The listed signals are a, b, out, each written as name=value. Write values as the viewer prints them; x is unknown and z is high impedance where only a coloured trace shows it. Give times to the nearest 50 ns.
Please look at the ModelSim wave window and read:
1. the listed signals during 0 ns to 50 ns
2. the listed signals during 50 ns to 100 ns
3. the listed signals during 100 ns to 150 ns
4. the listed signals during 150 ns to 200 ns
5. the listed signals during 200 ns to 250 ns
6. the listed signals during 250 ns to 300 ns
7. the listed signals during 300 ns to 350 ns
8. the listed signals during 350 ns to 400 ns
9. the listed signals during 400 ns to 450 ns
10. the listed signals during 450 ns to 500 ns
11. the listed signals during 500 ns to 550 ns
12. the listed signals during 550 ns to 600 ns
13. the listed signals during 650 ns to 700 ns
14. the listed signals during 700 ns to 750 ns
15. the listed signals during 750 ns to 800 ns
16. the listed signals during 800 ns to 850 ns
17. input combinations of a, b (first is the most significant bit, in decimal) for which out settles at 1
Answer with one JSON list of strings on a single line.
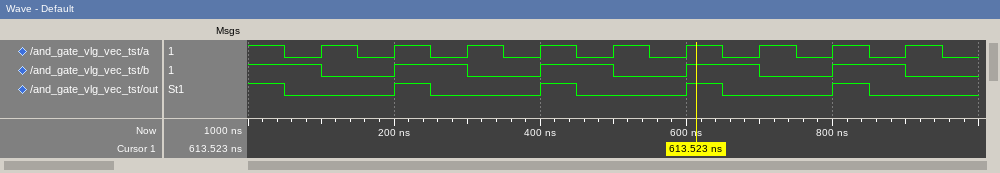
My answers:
["a=1, b=1, out=1", "a=0, b=1, out=0", "a=1, b=0, out=0", "a=0, b=0, out=0", "a=1, b=1, out=1", "a=0, b=1, out=0", "a=1, b=0, out=0", "a=0, b=0, out=0", "a=1, b=1, out=1", "a=0, b=1, out=0", "a=1, b=0, out=0", "a=0, b=0, out=0", "a=0, b=1, out=0", "a=1, b=0, out=0", "a=0, b=0, out=0", "a=1, b=1, out=1", "3"]
